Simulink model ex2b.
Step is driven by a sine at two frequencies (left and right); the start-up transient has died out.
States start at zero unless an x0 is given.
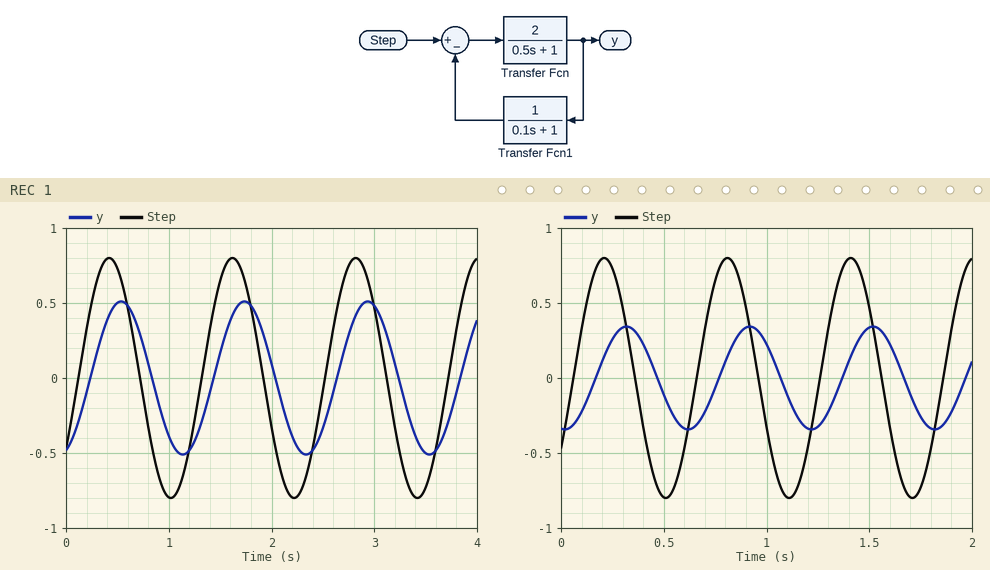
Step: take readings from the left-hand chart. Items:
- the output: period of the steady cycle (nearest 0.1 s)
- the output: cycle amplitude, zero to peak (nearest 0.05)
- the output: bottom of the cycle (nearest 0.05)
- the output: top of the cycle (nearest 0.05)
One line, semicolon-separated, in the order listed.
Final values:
1.2 s; 0.50; -0.50; 0.50
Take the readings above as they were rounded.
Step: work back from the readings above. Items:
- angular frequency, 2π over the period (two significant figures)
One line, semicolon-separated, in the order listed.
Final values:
5.2 rad/s
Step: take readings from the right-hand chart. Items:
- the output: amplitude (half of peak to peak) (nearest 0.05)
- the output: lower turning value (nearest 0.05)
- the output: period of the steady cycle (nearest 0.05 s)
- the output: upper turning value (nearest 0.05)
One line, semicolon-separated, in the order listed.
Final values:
0.35; -0.35; 0.60 s; 0.35
